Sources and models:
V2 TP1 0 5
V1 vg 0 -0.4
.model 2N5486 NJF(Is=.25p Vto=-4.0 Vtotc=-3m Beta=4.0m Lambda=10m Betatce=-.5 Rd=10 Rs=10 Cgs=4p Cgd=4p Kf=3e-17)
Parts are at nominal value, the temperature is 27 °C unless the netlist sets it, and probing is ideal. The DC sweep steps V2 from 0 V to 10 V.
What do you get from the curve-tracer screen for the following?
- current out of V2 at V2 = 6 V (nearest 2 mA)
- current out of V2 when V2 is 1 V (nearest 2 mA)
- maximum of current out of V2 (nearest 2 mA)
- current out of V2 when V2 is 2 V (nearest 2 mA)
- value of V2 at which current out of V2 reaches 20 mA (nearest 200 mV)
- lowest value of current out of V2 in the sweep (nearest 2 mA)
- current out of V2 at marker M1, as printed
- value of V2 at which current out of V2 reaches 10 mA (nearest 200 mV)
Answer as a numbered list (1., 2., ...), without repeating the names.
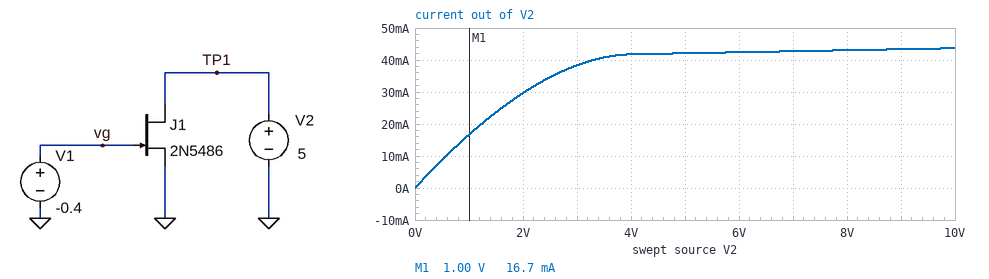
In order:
1. 42 mA
2. 16 mA
3. 44 mA
4. 30 mA
5. 1.2 V
6. 0 A
7. 16.7 mA
8. 600 mV
